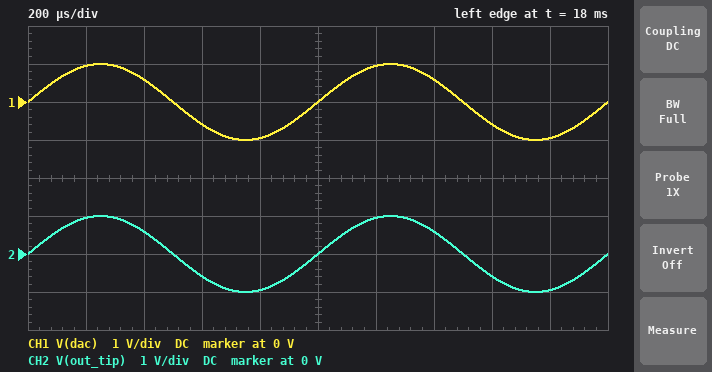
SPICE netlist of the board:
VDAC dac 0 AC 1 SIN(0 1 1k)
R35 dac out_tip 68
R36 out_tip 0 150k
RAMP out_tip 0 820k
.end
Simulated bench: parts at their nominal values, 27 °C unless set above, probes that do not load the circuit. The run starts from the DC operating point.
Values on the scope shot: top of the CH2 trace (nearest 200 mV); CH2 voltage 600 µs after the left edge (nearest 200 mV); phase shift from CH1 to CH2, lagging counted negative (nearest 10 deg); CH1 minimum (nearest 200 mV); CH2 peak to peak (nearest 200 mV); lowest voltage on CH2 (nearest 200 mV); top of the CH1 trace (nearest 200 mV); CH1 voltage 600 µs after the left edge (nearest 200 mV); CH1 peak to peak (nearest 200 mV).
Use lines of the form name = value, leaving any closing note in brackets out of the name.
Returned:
top of the CH2 trace = 1.0 V
CH2 voltage 600 µs after the left edge = -600 mV
phase shift from CH1 to CH2, lagging counted negative = 0 deg
CH1 minimum = -1.0 V
CH2 peak to peak = 2.0 V
lowest voltage on CH2 = -1.0 V
top of the CH1 trace = 1.0 V
CH1 voltage 600 µs after the left edge = -600 mV
CH1 peak to peak = 2.0 V
